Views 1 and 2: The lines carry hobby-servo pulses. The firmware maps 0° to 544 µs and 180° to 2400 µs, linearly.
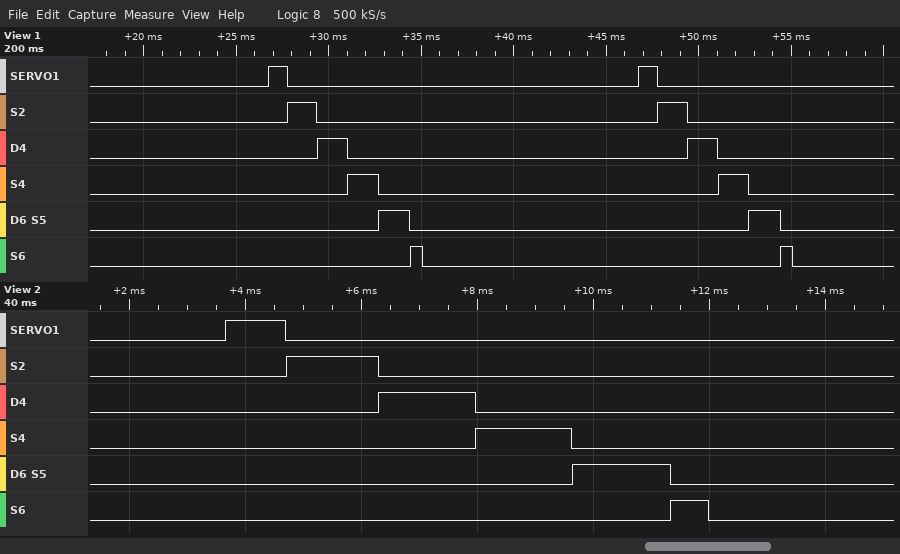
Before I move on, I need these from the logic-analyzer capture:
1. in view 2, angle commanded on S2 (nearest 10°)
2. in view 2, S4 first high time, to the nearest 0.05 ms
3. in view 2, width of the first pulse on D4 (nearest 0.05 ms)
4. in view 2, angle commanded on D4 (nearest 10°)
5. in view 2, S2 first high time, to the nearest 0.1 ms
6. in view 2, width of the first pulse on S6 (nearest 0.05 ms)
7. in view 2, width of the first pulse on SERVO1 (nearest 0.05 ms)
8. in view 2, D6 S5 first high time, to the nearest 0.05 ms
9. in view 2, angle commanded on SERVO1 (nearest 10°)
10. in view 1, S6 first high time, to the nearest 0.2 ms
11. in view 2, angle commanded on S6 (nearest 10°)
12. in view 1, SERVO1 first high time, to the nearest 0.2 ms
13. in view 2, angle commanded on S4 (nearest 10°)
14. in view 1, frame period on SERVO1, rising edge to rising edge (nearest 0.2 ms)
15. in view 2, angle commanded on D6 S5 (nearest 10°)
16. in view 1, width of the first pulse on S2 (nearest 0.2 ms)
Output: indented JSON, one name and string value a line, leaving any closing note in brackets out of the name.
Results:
{
  "in view 2, angle commanded on S2": "100°",
  "in view 2, S4 first high time, to the nearest 0.05 ms": "1.65 ms",
  "in view 2, width of the first pulse on D4": "1.65 ms",
  "in view 2, angle commanded on D4": "110°",
  "in view 2, S2 first high time, to the nearest 0.1 ms": "1.6 ms",
  "in view 2, width of the first pulse on S6": "0.65 ms",
  "in view 2, width of the first pulse on SERVO1": "1.05 ms",
  "in view 2, D6 S5 first high time, to the nearest 0.05 ms": "1.70 ms",
  "in view 2, angle commanded on SERVO1": "50°",
  "in view 1, S6 first high time, to the nearest 0.2 ms": "0.6 ms",
  "in view 2, angle commanded on S6": "10°",
  "in view 1, SERVO1 first high time, to the nearest 0.2 ms": "1.0 ms",
  "in view 2, angle commanded on S4": "110°",
  "in view 1, frame period on SERVO1, rising edge to rising edge": "20.0 ms",
  "in view 2, angle commanded on D6 S5": "110°",
  "in view 1, width of the first pulse on S2": "1.6 ms"
}
